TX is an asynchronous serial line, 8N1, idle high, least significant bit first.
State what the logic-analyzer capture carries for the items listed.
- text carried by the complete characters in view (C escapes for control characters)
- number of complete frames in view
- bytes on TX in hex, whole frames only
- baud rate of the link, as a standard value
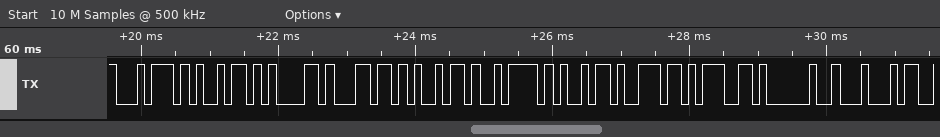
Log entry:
"tializing D"
11
74 69 61 6C 69 7A 69 6E 67 20 44
9600 baud
